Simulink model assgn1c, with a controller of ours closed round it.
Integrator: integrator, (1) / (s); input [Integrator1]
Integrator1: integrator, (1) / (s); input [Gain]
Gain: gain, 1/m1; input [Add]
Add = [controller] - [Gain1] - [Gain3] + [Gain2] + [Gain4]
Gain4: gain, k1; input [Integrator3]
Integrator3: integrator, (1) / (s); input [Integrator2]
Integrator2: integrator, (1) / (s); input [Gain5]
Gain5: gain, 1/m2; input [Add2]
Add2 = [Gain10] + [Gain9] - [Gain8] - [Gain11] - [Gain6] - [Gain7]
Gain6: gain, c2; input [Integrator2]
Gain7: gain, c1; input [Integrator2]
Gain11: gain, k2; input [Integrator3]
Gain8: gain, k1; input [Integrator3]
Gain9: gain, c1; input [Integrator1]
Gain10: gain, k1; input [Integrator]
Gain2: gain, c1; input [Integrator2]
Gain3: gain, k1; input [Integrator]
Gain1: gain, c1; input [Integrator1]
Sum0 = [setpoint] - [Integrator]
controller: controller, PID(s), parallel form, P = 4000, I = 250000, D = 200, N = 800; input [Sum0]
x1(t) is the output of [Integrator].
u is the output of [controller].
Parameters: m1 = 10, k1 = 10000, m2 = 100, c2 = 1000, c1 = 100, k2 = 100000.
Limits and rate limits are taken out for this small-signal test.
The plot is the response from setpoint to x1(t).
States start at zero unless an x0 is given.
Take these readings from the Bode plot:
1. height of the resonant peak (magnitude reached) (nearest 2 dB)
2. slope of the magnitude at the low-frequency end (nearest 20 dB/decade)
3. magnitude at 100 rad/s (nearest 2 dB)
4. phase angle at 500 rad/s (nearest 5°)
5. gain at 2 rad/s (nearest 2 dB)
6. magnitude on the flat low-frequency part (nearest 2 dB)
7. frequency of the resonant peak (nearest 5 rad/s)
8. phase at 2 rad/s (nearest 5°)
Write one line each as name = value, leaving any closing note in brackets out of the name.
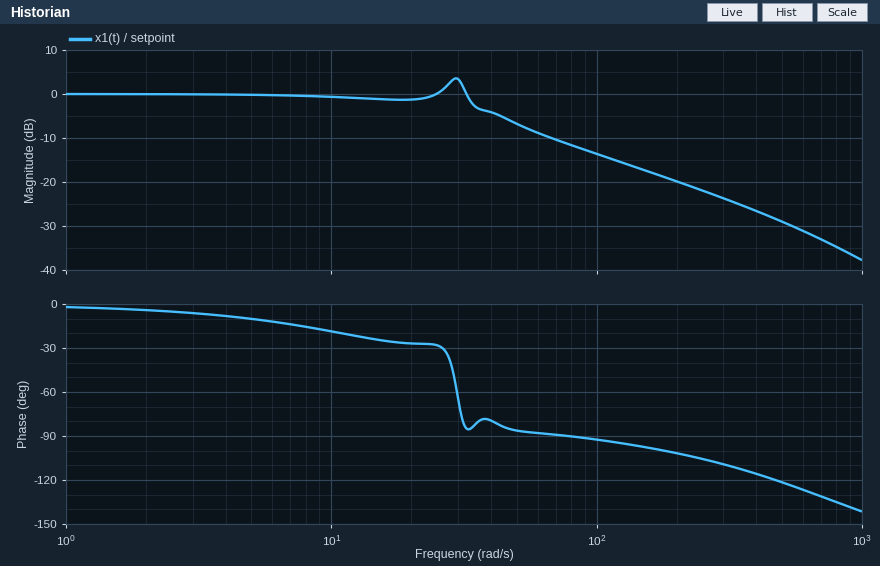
height of the resonant peak (magnitude reached) = 4 dB
slope of the magnitude at the low-frequency end = 0 dB/decade
magnitude at 100 rad/s = -14 dB
phase angle at 500 rad/s = -120°
gain at 2 rad/s = 0 dB
magnitude on the flat low-frequency part = 0 dB
frequency of the resonant peak = 30 rad/s
phase at 2 rad/s = -5°
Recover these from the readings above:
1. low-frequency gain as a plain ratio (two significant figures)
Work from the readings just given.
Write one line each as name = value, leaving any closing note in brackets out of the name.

low-frequency gain as a plain ratio = 1.0
